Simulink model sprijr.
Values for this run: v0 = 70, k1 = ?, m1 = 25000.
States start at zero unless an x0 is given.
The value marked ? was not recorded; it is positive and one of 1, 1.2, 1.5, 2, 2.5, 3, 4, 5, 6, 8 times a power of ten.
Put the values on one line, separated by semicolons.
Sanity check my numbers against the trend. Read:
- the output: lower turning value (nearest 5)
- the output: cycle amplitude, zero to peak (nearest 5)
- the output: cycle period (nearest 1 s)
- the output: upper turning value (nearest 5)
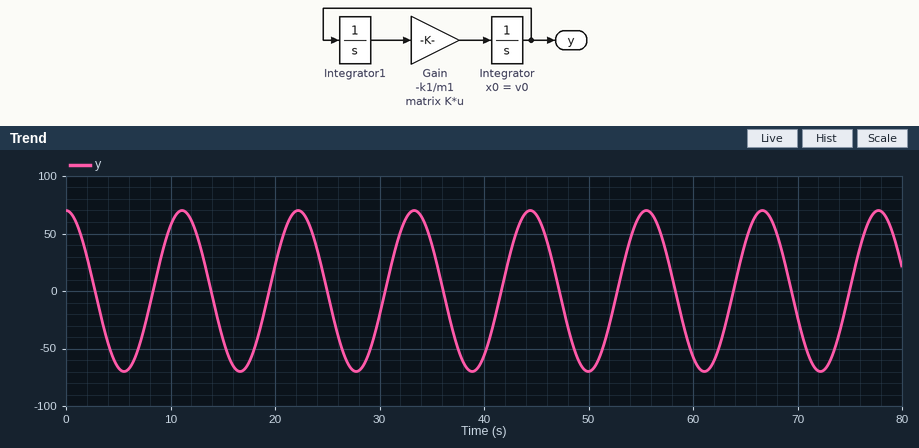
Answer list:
-70; 70; 11 s; 70
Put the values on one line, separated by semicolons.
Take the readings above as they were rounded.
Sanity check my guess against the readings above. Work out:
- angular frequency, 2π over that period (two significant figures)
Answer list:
0.57 rad/s
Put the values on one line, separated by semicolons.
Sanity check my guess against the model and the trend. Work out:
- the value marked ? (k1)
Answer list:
8000
